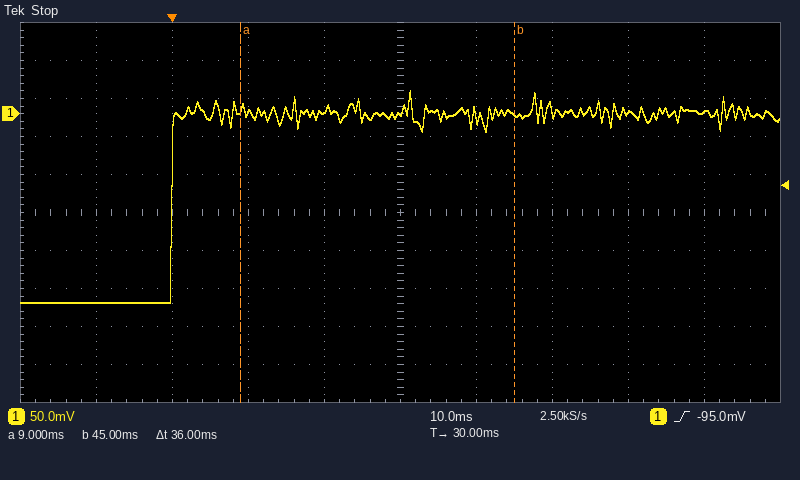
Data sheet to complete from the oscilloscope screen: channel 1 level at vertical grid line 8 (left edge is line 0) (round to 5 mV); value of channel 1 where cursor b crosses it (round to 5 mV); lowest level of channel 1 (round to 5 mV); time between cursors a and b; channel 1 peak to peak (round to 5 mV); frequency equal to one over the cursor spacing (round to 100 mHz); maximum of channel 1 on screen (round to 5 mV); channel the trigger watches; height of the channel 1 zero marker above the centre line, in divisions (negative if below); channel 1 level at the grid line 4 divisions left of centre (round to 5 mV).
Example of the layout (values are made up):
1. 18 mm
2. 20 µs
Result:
1. 0 mV
2. 0 mV
3. -250 mV
4. 36 ms
5. 280 mV
6. 27.8 Hz
7. 30 mV
8. channel 1
9. +2.6 div
10. -250 mV
